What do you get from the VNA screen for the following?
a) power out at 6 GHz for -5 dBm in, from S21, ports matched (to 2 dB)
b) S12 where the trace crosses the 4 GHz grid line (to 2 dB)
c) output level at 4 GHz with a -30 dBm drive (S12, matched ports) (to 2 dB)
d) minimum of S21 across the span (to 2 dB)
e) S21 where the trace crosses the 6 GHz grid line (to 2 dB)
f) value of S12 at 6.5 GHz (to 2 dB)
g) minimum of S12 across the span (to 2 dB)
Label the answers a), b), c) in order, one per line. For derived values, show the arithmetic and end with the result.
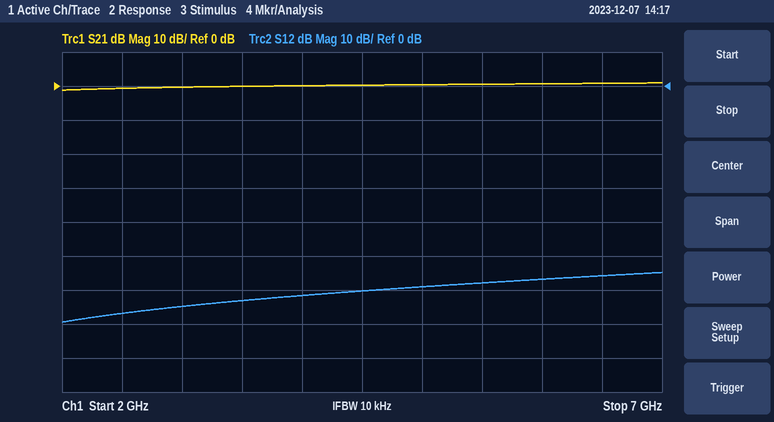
a) -5 dBm + (0 dB) = -4 dBm
b) -62 dB
c) -30 dBm + (-62 dB) = -92 dBm
d) -2 dB
e) 0 dB
f) -56 dB
g) -70 dB
